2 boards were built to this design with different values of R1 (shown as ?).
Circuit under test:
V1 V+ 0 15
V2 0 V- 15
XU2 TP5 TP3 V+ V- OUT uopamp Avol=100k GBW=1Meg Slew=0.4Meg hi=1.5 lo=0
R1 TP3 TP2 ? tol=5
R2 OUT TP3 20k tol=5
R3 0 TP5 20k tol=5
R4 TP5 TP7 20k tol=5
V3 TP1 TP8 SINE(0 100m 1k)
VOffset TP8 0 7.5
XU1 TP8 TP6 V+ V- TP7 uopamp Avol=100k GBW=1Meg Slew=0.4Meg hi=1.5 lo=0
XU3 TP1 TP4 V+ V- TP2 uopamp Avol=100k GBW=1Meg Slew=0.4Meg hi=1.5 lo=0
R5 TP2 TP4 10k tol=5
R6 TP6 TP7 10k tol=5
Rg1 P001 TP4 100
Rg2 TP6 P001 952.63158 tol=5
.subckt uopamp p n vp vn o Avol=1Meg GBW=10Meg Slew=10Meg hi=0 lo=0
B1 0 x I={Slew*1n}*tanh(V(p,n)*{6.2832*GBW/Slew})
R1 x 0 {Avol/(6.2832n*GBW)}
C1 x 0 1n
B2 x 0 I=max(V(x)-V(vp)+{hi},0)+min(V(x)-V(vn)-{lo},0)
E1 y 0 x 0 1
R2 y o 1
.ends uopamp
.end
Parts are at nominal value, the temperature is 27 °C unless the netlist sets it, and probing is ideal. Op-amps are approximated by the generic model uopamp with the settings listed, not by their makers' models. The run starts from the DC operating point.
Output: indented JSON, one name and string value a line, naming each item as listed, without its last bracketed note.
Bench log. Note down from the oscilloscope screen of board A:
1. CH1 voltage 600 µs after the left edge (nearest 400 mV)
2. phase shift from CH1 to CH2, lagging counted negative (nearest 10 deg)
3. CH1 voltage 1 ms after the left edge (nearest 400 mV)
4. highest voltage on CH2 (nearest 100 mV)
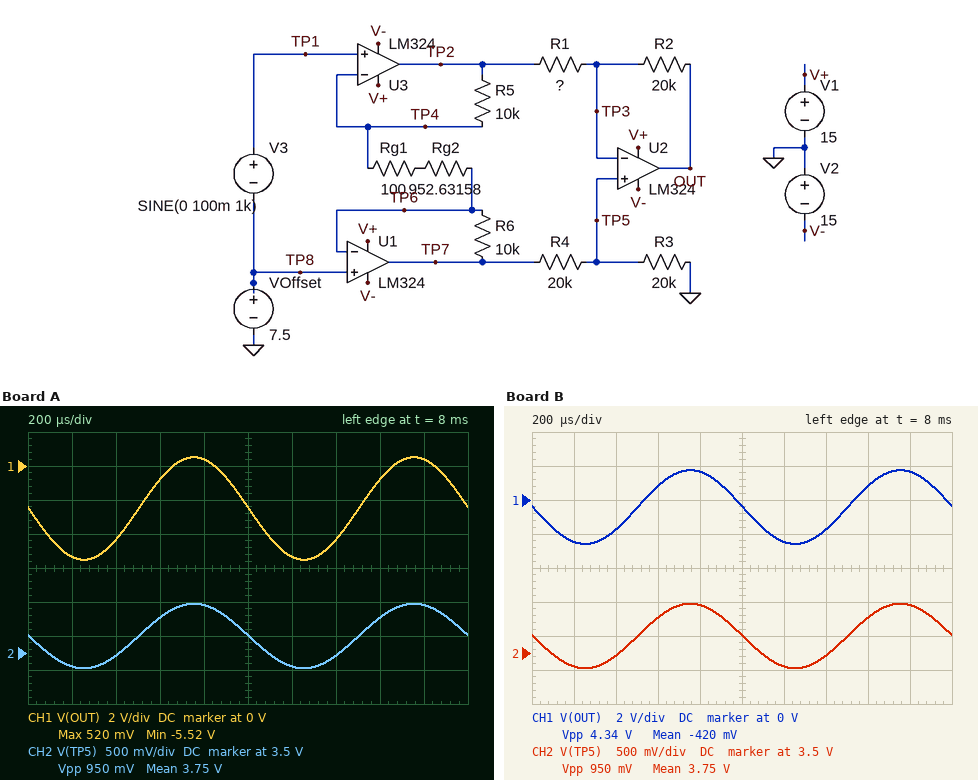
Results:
{
  "CH1 voltage 600 µs after the left edge": "-800 mV",
  "phase shift from CH1 to CH2, lagging counted negative": "0 deg",
  "CH1 voltage 1 ms after the left edge": "-2.4 V",
  "highest voltage on CH2": "4.2 V"
}
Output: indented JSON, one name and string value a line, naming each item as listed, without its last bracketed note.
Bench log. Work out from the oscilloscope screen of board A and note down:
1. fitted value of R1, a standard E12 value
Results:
{
  "fitted value of R1, a standard E12 value": "12 kΩ"
}
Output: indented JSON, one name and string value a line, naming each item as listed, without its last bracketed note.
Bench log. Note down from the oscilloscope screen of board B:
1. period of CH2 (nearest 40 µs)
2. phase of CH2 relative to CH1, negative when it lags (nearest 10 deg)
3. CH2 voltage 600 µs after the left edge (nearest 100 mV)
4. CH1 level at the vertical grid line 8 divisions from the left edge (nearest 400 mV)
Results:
{
  "period of CH2": "1.00 ms",
  "phase of CH2 relative to CH1, negative when it lags": "0 deg",
  "CH2 voltage 600 µs after the left edge": "4.0 V",
  "CH1 level at the vertical grid line 8 divisions from the left edge": "800 mV"
}
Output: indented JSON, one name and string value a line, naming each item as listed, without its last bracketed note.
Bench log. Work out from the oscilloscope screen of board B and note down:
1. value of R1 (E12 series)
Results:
{
  "value of R1": "18 kΩ"
}
